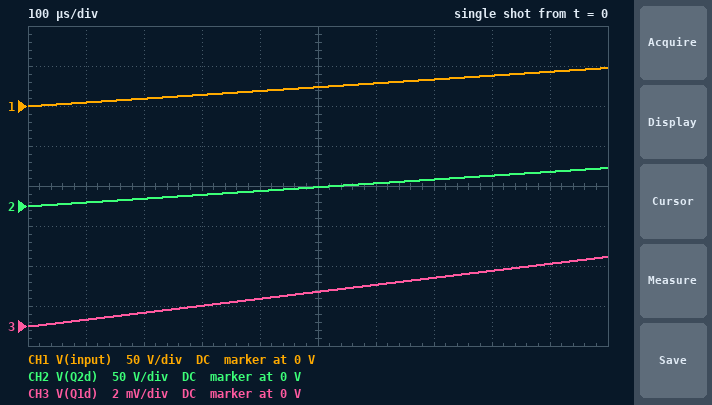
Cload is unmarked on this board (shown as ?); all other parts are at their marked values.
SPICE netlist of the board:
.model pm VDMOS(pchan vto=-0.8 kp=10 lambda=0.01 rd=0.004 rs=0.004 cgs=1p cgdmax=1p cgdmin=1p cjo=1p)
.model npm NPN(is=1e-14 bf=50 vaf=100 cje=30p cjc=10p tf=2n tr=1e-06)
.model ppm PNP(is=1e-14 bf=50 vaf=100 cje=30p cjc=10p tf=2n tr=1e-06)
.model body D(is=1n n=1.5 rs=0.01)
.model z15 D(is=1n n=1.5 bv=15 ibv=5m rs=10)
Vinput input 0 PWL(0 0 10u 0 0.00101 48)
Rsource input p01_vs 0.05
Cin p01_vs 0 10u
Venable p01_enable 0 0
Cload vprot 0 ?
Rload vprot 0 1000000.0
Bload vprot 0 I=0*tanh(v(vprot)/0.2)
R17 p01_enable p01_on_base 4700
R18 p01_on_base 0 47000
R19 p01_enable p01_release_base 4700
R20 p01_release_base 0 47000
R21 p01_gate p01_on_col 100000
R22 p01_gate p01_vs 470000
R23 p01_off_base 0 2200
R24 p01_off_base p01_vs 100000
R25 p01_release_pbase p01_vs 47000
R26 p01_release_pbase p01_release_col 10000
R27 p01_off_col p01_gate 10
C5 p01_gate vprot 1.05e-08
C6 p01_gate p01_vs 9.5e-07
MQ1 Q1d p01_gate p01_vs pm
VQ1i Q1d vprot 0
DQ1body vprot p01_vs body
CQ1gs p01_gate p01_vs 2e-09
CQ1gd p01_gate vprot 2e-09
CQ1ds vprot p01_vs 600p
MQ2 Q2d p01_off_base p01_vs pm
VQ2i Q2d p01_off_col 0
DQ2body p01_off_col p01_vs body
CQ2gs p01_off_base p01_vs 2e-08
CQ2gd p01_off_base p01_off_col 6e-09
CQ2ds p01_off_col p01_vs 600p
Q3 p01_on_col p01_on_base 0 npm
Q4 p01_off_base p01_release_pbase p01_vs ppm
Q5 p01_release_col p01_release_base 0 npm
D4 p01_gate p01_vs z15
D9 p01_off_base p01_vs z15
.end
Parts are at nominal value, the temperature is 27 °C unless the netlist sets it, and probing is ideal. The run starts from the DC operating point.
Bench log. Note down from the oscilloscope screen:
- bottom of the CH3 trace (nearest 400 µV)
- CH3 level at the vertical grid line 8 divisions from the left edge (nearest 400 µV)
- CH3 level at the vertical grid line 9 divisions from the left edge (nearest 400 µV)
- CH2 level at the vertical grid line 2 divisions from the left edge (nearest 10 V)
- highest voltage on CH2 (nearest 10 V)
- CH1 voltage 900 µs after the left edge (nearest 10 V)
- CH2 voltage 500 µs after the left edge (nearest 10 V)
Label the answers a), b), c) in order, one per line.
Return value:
a) 0 V
b) 2.8 mV
c) 3.2 mV
d) 10 V
e) 50 V
f) 40 V
g) 20 V
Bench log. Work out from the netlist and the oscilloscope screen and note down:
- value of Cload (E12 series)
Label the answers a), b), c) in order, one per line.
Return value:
a) 180 µF
